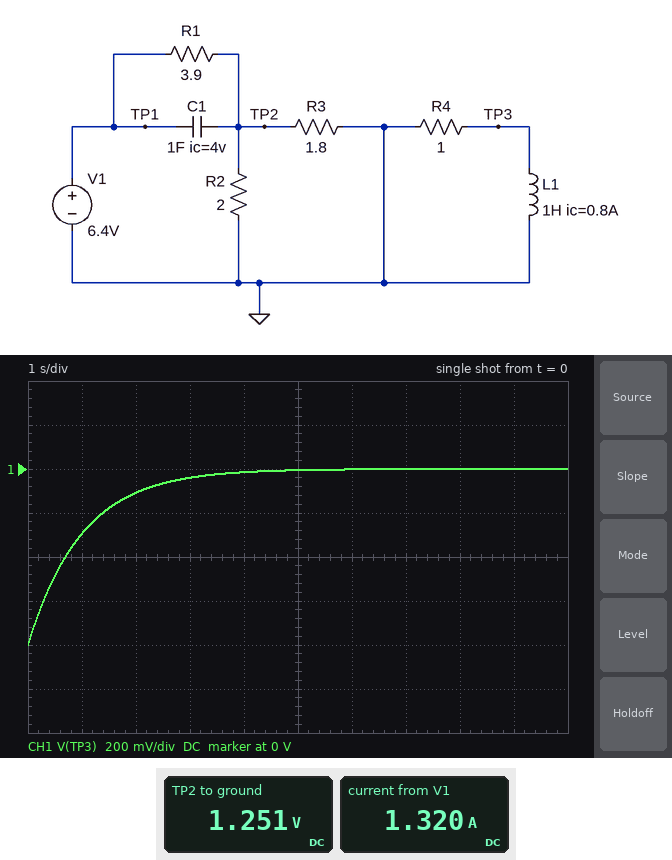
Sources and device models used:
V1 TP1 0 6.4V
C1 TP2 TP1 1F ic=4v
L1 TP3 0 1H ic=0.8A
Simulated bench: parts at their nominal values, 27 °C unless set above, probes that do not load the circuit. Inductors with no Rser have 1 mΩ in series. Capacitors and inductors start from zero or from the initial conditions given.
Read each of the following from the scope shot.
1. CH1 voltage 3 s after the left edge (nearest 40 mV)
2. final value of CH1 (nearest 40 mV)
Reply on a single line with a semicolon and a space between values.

-40 mV; 0 V
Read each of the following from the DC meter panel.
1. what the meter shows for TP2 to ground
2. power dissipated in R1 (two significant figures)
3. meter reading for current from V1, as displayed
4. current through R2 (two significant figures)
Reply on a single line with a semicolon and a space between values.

1.251 V; 6.8 W; 1.320 A; 630 mA
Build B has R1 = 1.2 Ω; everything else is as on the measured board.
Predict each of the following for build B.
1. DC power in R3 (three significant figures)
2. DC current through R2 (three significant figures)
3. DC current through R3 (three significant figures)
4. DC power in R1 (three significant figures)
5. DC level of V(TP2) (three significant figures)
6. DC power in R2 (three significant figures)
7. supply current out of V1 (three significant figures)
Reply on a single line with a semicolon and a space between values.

4.43 W; 1.41 A; 1.57 A; 10.7 W; 2.82 V; 3.99 W; 2.98 A
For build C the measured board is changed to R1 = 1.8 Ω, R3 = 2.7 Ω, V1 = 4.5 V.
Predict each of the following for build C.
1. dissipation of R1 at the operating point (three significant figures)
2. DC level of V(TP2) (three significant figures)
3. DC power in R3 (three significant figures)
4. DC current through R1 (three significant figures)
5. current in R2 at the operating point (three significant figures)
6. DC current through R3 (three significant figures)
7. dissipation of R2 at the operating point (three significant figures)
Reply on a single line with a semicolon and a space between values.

4.19 W; 1.75 V; 1.14 W; 1.53 A; 877 mA; 649 mA; 1.54 W
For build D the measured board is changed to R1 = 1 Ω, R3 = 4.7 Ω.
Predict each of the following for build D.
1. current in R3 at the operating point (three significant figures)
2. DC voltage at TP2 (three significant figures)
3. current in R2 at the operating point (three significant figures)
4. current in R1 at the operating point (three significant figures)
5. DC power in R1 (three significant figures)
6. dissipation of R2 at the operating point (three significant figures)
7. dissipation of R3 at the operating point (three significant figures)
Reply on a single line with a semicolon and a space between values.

795 mA; 3.74 V; 1.87 A; 2.66 A; 7.09 W; 6.98 W; 2.97 W
